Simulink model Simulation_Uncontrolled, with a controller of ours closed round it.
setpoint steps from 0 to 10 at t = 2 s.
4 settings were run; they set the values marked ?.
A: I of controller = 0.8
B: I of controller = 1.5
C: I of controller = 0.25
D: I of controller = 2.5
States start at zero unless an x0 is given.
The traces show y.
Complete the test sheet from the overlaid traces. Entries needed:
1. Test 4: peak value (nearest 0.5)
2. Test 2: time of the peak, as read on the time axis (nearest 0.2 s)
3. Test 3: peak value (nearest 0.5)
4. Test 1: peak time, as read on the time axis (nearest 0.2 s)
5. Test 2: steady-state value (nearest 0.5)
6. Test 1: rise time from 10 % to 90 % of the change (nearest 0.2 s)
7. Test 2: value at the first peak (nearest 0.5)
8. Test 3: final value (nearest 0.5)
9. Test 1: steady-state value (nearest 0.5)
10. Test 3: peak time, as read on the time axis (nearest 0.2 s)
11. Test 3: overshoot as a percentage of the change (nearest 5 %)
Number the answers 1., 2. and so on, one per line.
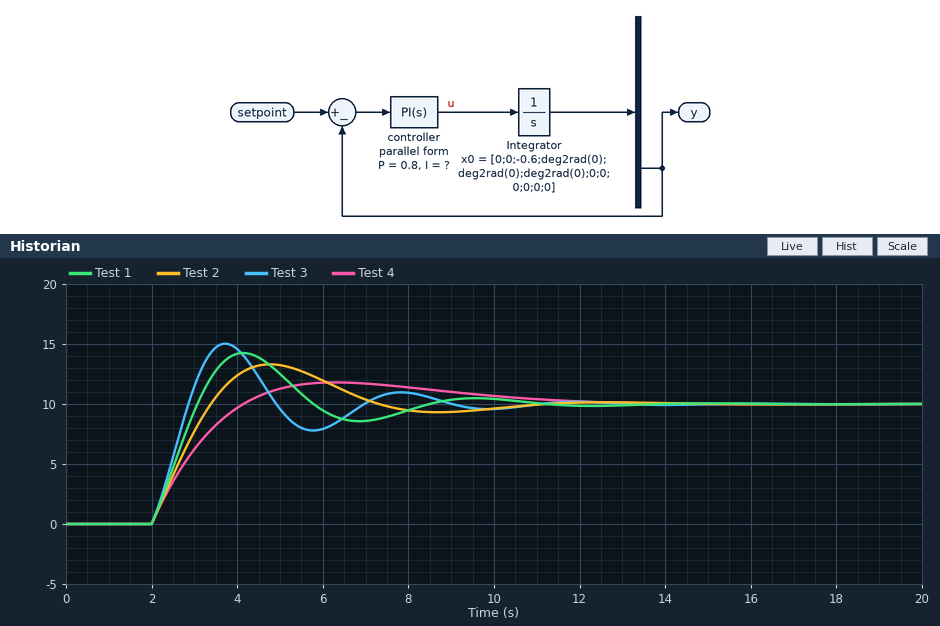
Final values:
1. 12.0
2. 4.8 s
3. 15.0
4. 4.2 s
5. 10.0
6. 0.8 s
7. 13.5
8. 10.0
9. 10.0
10. 3.8 s
11. 50 %
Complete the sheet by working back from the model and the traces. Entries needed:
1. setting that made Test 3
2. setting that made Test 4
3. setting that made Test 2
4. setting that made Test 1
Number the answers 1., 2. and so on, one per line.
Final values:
1. D
2. C
3. A
4. B
